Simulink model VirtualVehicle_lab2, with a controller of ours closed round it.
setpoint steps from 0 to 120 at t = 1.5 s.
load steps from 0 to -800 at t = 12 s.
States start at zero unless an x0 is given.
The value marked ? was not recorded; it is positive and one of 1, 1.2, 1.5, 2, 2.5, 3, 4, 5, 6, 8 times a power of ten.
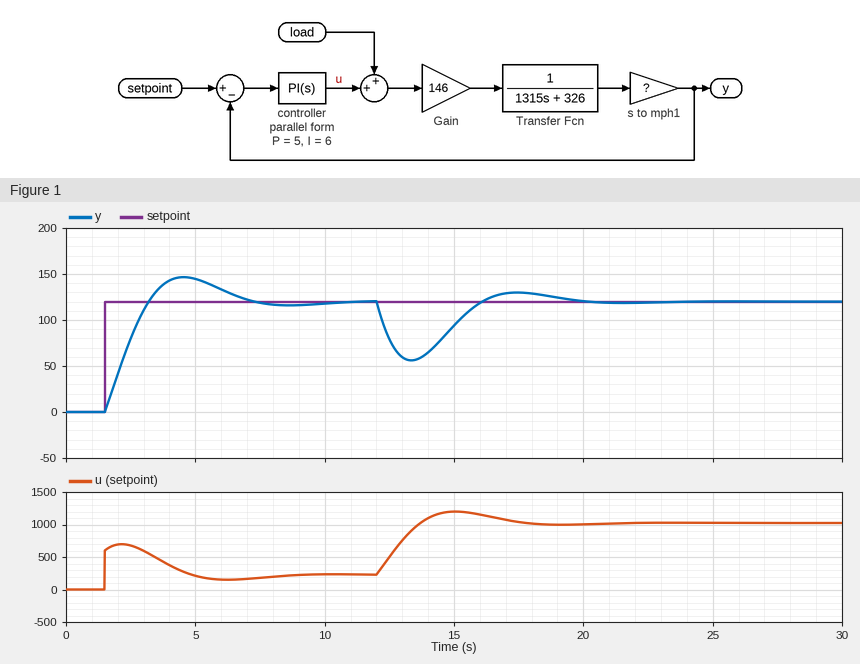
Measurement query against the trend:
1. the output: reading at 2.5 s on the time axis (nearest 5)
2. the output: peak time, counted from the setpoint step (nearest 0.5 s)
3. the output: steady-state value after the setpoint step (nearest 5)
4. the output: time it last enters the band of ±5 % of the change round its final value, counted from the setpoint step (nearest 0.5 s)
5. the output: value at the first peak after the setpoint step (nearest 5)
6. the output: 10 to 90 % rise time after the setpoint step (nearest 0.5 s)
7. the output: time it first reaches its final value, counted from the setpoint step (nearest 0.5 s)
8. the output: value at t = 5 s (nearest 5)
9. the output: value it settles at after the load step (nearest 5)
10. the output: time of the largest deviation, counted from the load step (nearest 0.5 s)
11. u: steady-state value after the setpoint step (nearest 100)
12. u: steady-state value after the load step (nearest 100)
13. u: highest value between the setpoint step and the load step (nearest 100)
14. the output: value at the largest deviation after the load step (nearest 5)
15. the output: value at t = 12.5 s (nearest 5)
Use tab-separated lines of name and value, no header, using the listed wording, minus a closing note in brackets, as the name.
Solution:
the output: reading at 2.5 s on the time axis	80
the output: peak time, counted from the setpoint step	3.0 s
the output: steady-state value after the setpoint step	120
the output: time it last enters the band of ±5 % of the change round its final value, counted from the setpoint step	5.0 s
the output: value at the first peak after the setpoint step	145
the output: 10 to 90 % rise time after the setpoint step	1.5 s
the output: time it first reaches its final value, counted from the setpoint step	1.5 s
the output: value at t = 5 s	145
the output: value it settles at after the load step	120
the output: time of the largest deviation, counted from the load step	1.5 s
u: steady-state value after the setpoint step	200
u: steady-state value after the load step	1000
u: highest value between the setpoint step and the load step	700
the output: value at the largest deviation after the load step	55
the output: value at t = 12.5 s	80
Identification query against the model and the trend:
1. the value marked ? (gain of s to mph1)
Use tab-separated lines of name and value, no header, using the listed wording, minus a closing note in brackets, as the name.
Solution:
the value marked ?	1.2
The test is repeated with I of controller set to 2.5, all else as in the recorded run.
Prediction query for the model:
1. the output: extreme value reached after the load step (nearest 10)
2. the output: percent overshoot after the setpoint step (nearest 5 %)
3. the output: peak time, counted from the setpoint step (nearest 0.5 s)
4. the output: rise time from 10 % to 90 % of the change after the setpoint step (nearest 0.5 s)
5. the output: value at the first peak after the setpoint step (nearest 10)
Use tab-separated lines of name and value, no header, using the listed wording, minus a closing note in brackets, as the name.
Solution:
the output: extreme value reached after the load step	40
the output: percent overshoot after the setpoint step	10 %
the output: peak time, counted from the setpoint step	5.0 s
the output: rise time from 10 % to 90 % of the change after the setpoint step	2.0 s
the output: value at the first peak after the setpoint step	130
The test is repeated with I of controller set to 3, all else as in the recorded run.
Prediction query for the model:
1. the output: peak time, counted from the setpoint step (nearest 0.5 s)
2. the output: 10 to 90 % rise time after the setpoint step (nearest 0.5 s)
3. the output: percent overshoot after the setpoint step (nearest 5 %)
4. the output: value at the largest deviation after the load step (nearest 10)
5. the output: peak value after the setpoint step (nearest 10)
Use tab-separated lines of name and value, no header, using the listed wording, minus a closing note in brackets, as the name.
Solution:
the output: peak time, counted from the setpoint step	4.5 s
the output: 10 to 90 % rise time after the setpoint step	2.0 s
the output: percent overshoot after the setpoint step	10 %
the output: value at the largest deviation after the load step	40
the output: peak value after the setpoint step	130
